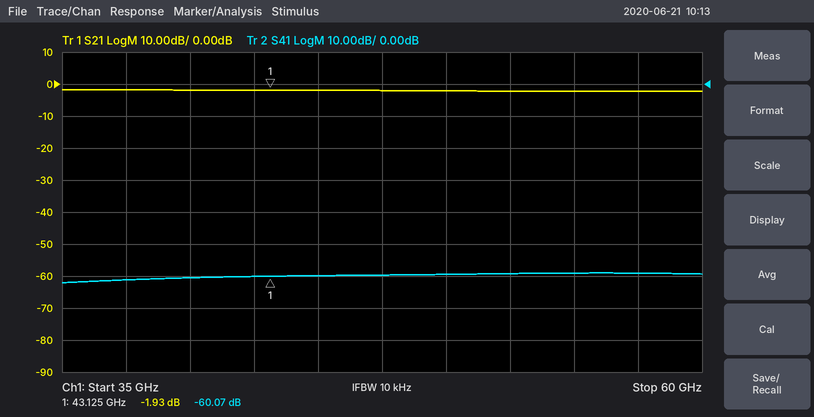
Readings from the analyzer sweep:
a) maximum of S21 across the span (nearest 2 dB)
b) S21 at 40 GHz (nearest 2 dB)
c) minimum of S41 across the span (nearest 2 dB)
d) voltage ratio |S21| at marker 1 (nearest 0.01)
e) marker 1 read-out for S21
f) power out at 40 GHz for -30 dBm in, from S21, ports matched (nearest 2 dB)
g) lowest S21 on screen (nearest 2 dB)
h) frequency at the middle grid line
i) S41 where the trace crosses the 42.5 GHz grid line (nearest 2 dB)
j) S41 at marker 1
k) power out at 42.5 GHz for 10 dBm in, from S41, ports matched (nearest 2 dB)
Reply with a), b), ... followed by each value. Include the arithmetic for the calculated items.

a) -2 dB
b) -2 dB
c) -62 dB
d) 10^(-1.93/20) ≈ 0.80
e) -1.93 dB
f) -30 dBm + (-2 dB) = -32 dBm
g) -2 dB
h) 47.5 GHz
i) -60 dB
j) -60.07 dB
k) 10 dBm + (-60 dB) = -50 dBm
